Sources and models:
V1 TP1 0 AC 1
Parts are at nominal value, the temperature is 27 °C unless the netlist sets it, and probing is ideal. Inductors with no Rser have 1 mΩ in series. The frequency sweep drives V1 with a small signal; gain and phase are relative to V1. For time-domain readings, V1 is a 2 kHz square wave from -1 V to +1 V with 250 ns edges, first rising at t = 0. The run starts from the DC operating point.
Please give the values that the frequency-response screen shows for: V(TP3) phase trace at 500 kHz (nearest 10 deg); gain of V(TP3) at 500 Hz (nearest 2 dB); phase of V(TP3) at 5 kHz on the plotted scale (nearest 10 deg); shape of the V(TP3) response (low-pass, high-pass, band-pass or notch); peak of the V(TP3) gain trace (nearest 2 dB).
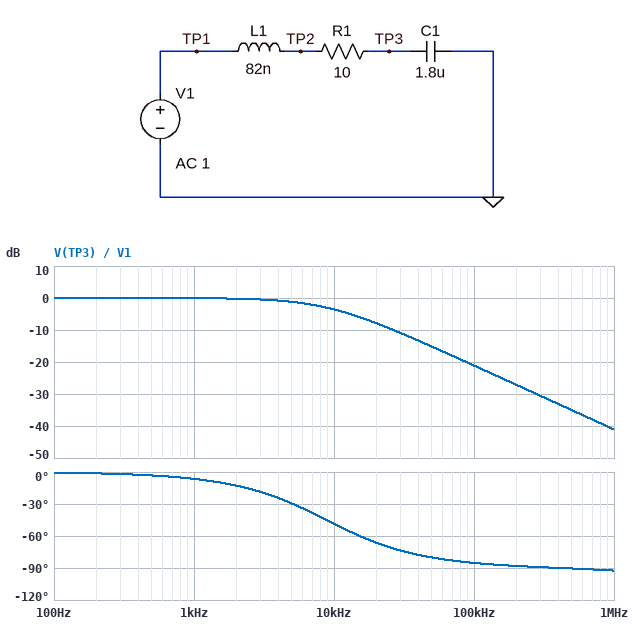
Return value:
-90 deg
0 dB
-30 deg
low-pass
0 dB
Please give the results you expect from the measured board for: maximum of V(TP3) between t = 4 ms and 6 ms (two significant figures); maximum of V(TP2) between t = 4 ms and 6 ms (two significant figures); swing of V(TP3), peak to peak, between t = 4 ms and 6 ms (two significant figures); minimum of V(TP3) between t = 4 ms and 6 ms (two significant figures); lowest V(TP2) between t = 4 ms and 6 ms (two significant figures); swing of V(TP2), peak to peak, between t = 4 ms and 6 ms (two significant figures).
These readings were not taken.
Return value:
1.0 V
1.0 V
2.0 V
-1.0 V
-1.0 V
2.0 V
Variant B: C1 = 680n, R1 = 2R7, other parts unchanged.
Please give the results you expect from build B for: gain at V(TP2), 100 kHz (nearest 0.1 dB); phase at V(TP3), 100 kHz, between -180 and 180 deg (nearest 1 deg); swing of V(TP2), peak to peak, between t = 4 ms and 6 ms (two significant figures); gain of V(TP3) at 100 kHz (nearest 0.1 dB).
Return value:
0.1 dB
-50 deg
2.1 V
-3.6 dB
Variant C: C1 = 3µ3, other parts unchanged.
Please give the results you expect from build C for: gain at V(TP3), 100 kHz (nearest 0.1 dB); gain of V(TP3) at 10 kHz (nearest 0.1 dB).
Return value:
-26.3 dB
-7.2 dB
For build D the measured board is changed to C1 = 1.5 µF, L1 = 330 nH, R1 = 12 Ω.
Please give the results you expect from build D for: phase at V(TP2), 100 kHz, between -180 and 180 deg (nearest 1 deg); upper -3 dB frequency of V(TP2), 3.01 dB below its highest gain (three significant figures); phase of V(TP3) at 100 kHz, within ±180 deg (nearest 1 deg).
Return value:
-1 deg
5.78 MHz
-86 deg
